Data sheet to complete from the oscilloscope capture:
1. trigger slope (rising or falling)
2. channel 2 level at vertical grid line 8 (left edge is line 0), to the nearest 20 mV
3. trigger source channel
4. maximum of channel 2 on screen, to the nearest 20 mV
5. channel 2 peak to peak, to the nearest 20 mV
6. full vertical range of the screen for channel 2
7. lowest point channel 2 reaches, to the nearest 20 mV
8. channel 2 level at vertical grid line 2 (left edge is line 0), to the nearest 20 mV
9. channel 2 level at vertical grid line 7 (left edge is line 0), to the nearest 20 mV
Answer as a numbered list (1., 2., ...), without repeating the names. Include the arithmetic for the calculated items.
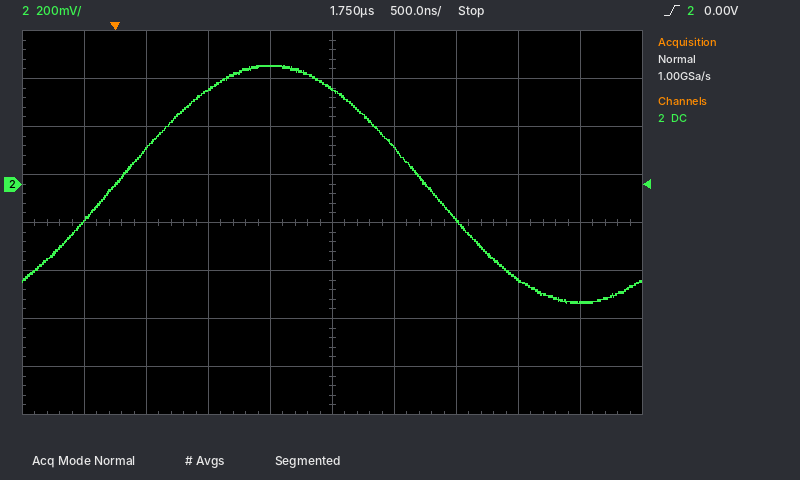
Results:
1. rising
2. -400 mV
3. channel 2
4. 500 mV
5. 500 mV − (-500 mV) = 1.00 V
6. 1.6 V
7. -500 mV
8. 140 mV
9. -160 mV
